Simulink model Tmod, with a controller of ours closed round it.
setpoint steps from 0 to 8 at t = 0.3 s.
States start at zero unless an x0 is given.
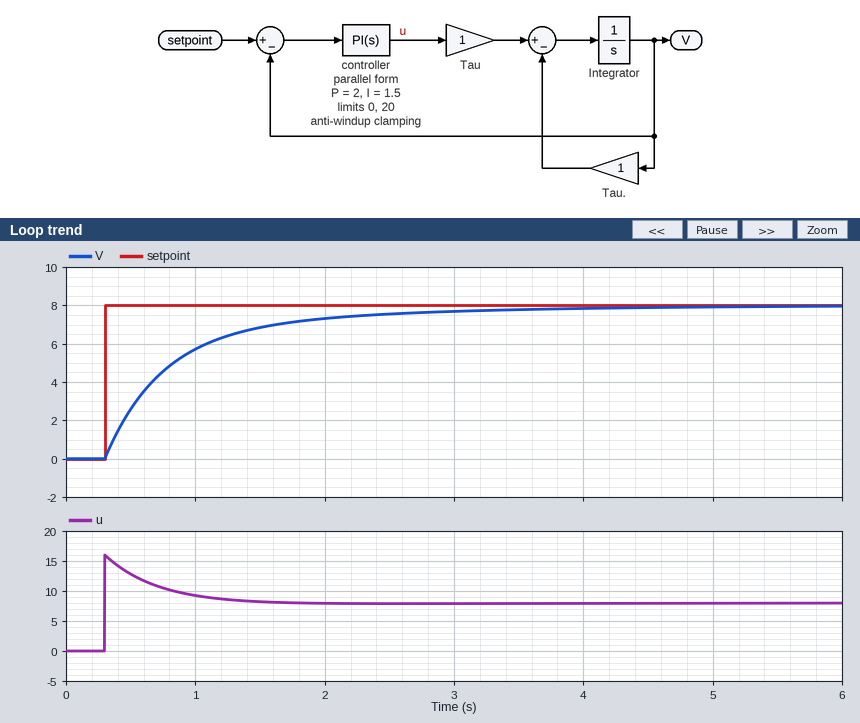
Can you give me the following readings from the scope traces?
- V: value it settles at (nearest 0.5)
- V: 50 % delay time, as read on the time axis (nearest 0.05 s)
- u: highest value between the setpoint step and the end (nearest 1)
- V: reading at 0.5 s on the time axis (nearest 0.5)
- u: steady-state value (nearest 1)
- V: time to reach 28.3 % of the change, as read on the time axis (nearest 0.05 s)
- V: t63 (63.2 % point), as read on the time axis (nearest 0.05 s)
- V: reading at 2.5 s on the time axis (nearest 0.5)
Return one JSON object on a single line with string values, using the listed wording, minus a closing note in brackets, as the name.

{"V: value it settles at": "8.0", "V: 50 % delay time, as read on the time axis": "0.65 s", "u: highest value between the setpoint step and the end": "16", "V: reading at 0.5 s on the time axis": "2.5", "u: steady-state value": "8", "V: time to reach 28.3 % of the change, as read on the time axis": "0.45 s", "V: t63 (63.2 % point), as read on the time axis": "0.85 s", "V: reading at 2.5 s on the time axis": "7.5"}
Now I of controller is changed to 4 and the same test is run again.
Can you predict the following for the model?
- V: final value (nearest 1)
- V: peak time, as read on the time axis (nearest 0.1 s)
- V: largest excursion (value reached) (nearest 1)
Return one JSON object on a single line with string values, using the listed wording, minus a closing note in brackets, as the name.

{"V: final value": "8", "V: peak time, as read on the time axis": "1.8 s", "V: largest excursion (value reached)": "9"}
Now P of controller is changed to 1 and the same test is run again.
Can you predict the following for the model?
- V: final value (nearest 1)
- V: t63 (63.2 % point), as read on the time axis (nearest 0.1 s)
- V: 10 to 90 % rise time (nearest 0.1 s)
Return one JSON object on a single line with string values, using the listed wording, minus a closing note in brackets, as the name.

{"V: final value": "8", "V: t63 (63.2 % point), as read on the time axis": "1.1 s", "V: 10 to 90 % rise time": "1.4 s"}
